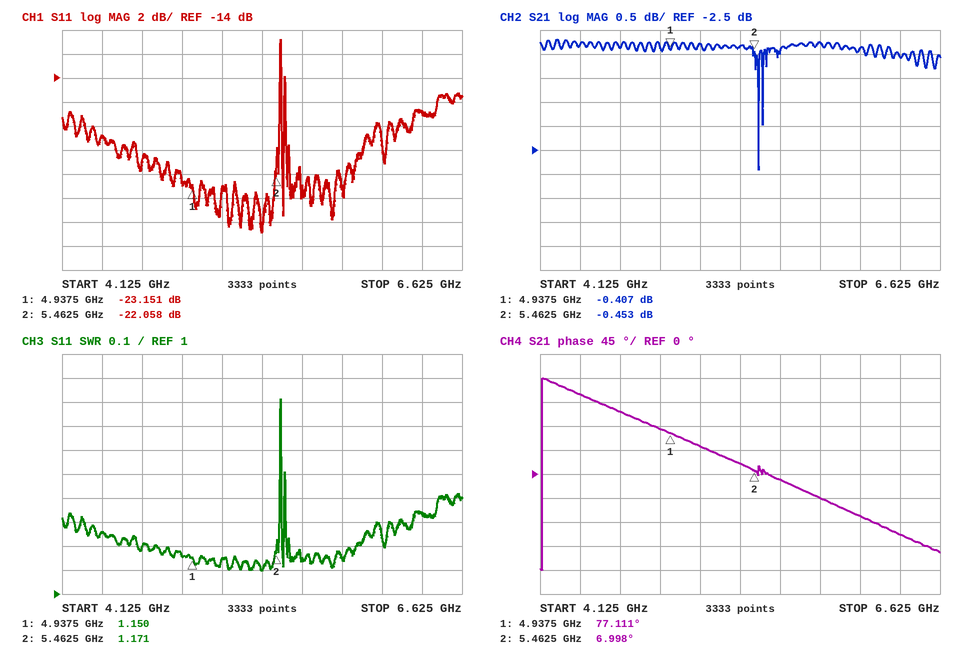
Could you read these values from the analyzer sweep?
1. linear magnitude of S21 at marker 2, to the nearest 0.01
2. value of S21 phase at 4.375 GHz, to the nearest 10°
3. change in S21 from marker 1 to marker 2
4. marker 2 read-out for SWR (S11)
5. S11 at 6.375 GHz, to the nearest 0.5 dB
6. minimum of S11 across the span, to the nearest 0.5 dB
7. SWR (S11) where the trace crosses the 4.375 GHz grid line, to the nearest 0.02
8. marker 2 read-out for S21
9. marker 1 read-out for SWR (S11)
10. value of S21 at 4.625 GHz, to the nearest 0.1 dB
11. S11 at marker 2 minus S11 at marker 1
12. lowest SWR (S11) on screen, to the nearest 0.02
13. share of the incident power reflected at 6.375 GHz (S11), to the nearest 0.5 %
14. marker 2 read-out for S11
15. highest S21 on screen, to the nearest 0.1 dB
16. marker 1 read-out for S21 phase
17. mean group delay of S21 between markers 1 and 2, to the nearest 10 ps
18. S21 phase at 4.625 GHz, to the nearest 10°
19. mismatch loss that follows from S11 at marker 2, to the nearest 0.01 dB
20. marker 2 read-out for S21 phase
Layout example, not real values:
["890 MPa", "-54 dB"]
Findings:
["0.95", "150°", "-0.046 dB", "1.171", "-17.0 dB", "-27.0 dB", "1.26", "-0.453 dB", "1.150", "-0.4 dB", "1.093 dB", "1.10", "2.0 %", "-22.058 dB", "-0.2 dB", "77.111°", "370 ps", "120°", "0.03 dB", "6.998°"]
